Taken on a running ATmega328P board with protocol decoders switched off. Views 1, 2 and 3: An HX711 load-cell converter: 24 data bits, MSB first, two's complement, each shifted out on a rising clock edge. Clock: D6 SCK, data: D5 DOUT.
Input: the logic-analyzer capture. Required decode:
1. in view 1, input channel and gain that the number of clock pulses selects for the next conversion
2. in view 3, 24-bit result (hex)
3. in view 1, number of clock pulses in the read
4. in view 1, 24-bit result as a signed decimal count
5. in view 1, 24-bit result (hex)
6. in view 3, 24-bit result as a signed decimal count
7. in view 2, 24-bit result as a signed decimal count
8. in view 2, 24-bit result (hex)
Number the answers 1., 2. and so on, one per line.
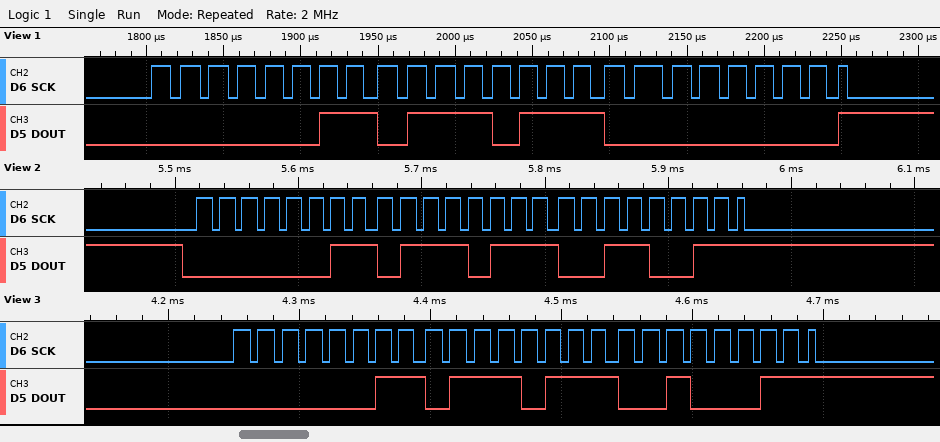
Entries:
1. channel A, gain 128
2. 0x037723
3. 25
4. 227072
5. 0x037700
6. 227107
7. 227123
8. 0x037733
